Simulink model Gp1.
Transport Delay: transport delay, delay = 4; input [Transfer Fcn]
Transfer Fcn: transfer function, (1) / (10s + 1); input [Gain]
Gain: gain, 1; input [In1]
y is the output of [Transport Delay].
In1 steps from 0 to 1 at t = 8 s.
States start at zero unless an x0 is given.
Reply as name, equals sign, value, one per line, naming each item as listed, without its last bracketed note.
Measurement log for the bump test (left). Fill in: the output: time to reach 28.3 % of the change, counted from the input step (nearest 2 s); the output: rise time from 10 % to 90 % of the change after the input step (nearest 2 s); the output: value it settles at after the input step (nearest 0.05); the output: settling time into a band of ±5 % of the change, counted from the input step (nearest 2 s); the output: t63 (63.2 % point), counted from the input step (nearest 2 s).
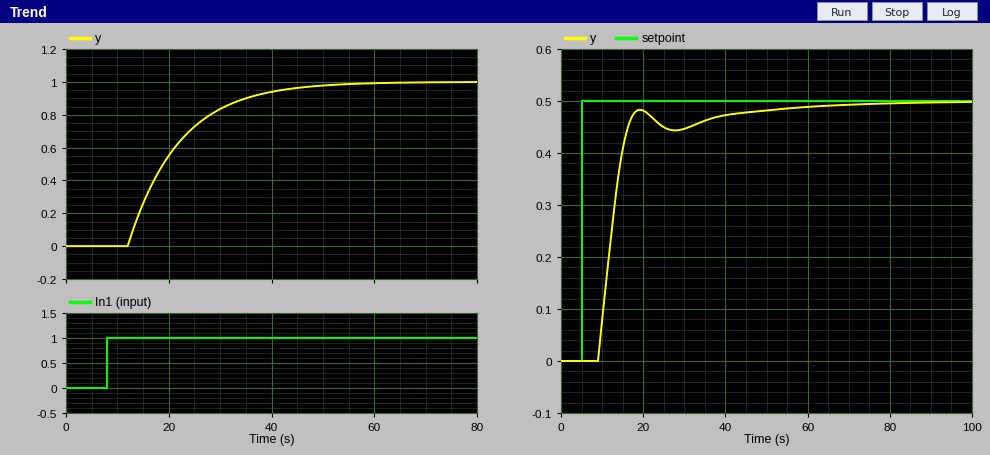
the output: time to reach 28.3 % of the change, counted from the input step = 8 s
the output: rise time from 10 % to 90 % of the change after the input step = 22 s
the output: value it settles at after the input step = 1.00
the output: settling time into a band of ±5 % of the change, counted from the input step = 34 s
the output: t63 (63.2 % point), counted from the input step = 14 s
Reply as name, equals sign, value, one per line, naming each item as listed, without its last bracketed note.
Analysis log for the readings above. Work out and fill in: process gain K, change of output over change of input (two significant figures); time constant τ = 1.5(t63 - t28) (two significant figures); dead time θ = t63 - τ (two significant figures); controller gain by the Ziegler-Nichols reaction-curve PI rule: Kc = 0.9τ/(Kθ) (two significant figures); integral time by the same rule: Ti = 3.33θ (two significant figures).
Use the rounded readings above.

process gain K, change of output over change of input = 1.0
time constant τ = 1.5(t63 - t28) = 9.0 s
dead time θ = t63 - τ = 5.0 s
controller gain by the Ziegler-Nichols reaction-curve PI rule: Kc = 0.9τ/(Kθ) = 1.6
integral time by the same rule: Ti = 3.33θ = 17 s
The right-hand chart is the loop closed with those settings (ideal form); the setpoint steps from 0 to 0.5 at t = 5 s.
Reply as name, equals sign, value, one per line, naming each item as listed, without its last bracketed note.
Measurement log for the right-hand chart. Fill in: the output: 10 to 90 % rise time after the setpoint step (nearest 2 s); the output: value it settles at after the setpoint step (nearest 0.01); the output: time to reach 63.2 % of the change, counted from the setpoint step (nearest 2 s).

the output: 10 to 90 % rise time after the setpoint step = 6 s
the output: value it settles at after the setpoint step = 0.50
the output: time to reach 63.2 % of the change, counted from the setpoint step = 8 s
